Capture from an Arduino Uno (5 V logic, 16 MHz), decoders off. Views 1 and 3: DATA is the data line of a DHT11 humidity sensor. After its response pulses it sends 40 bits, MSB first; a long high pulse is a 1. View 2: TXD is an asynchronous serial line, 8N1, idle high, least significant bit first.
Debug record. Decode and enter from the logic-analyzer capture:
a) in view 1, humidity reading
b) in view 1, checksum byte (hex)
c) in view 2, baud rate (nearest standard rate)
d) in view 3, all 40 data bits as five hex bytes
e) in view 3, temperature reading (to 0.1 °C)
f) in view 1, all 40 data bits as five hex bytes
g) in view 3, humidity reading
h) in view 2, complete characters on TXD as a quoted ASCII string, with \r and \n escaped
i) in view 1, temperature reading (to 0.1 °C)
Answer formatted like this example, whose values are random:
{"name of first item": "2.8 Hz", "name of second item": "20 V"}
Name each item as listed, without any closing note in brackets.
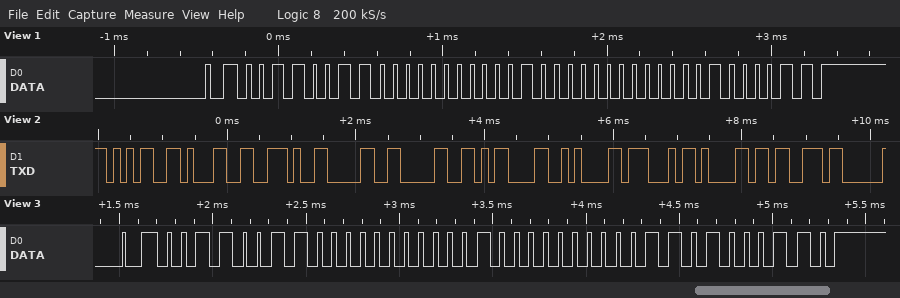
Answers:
{"in view 1, humidity reading": "51 %", "in view 1, checksum byte": "0x43", "in view 2, baud rate": "9600 baud", "in view 3, all 40 data bits as five hex bytes": "33 00 10 03 46", "in view 3, temperature reading": "16.3 °C", "in view 1, all 40 data bits as five hex bytes": "33 00 10 00 43", "in view 3, humidity reading": "51 %", "in view 2, complete characters on TXD as a quoted ASCII string, with \\r and \\n escaped": "\"51.00\\r\\nGas\"", "in view 1, temperature reading": "16.0 °C"}
